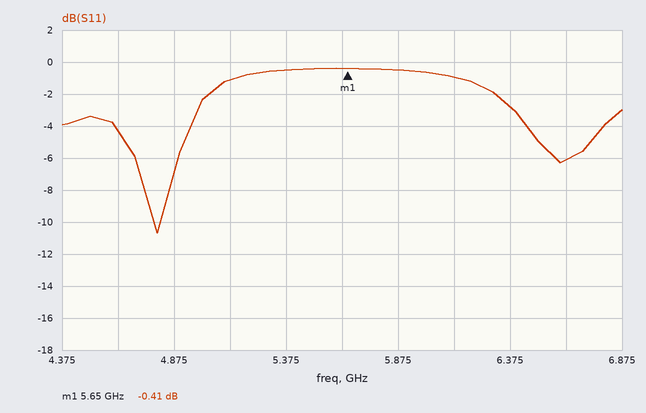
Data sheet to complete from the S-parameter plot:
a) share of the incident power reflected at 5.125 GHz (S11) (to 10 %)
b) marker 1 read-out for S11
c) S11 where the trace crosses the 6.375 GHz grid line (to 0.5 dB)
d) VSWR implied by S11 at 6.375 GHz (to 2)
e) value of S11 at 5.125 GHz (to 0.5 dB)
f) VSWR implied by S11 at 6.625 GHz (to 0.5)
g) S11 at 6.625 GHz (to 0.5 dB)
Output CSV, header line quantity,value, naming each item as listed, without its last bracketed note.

quantity,value
share of the incident power reflected at 5.125 GHz (S11),80 %
marker 1 read-out for S11,-0.41 dB
S11 where the trace crosses the 6.375 GHz grid line,-3.0 dB
VSWR implied by S11 at 6.375 GHz,6
value of S11 at 5.125 GHz,-1.0 dB
VSWR implied by S11 at 6.625 GHz,3.0
S11 at 6.625 GHz,-6.0 dB
